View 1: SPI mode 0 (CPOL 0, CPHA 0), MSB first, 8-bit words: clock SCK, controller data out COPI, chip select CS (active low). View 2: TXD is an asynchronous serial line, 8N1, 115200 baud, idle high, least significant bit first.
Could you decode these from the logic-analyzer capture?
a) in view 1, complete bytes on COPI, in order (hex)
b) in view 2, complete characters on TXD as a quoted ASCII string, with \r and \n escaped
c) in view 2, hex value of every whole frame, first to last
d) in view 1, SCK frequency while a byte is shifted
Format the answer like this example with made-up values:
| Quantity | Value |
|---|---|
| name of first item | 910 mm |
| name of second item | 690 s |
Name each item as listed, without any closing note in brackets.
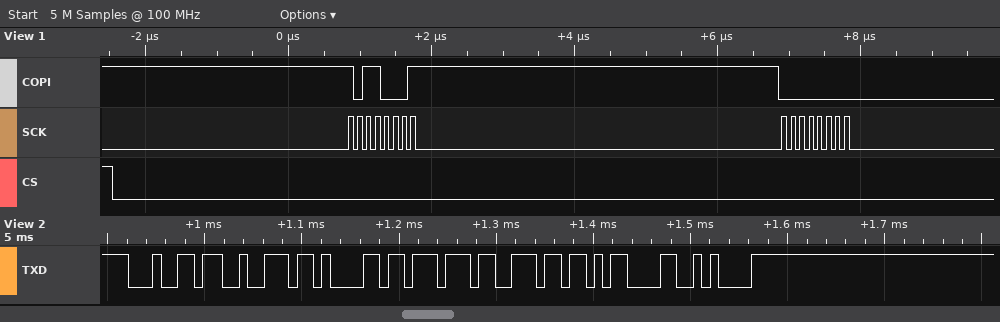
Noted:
| Quantity | Value |
|---|---|
| in view 1, complete bytes on COPI, in order | B1 00 |
| in view 2, complete characters on TXD as a quoted ASCII string, with \r and \n escaped | "drawn\r\n" |
| in view 2, hex value of every whole frame, first to last | 64 72 61 77 6E 0D 0A |
| in view 1, SCK frequency while a byte is shifted | 8 MHz |
